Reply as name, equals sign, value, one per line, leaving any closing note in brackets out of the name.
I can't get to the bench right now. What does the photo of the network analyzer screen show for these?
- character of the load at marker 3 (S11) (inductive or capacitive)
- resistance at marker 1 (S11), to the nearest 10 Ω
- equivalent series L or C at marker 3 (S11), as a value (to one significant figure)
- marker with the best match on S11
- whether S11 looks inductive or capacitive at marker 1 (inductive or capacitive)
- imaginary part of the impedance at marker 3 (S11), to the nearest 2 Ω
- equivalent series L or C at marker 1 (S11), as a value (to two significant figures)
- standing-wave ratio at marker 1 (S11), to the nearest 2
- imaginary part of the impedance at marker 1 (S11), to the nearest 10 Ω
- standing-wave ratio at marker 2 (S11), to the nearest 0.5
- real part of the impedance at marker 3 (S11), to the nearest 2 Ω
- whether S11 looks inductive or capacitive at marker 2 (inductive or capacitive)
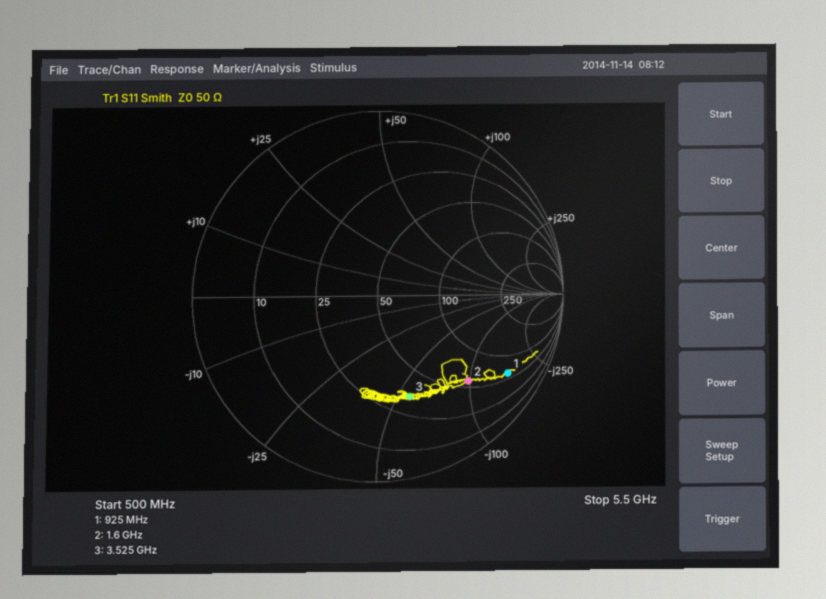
character of the load at marker 3 (S11) = capacitive
resistance at marker 1 (S11), to the nearest 10 Ω = 60 Ω
equivalent series L or C at marker 3 (S11), as a value = 800 fF
marker with the best match on S11 = marker 3
whether S11 looks inductive or capacitive at marker 1 = capacitive
imaginary part of the impedance at marker 3 (S11), to the nearest 2 Ω = -56 Ω
equivalent series L or C at marker 1 (S11), as a value = 1.1 pF
standing-wave ratio at marker 1 (S11), to the nearest 2 = 10
imaginary part of the impedance at marker 1 (S11), to the nearest 10 Ω = -160 Ω
standing-wave ratio at marker 2 (S11), to the nearest 0.5 = 5.0
real part of the impedance at marker 3 (S11), to the nearest 2 Ω = 34 Ω
whether S11 looks inductive or capacitive at marker 2 = capacitive
